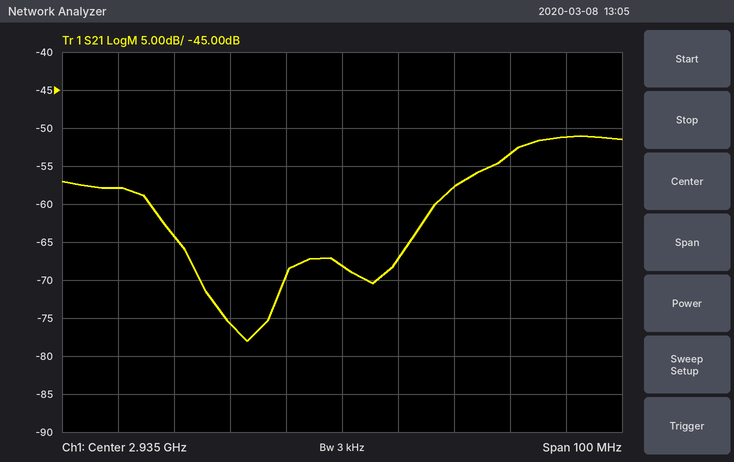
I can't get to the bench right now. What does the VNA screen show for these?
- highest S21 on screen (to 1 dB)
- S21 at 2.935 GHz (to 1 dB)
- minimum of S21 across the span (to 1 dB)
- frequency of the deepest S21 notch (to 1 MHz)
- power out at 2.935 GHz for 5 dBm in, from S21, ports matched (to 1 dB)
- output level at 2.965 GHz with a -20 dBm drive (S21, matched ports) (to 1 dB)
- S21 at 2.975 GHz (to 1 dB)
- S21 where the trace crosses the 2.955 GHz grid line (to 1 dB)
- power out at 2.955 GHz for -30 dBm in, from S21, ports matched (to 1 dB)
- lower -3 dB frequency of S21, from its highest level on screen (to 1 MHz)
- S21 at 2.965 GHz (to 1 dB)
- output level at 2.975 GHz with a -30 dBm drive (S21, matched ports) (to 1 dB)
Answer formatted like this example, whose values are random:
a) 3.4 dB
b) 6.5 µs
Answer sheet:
a) -51 dB
b) -68 dB
c) -78 dB
d) 2.918 GHz
e) -63 dBm
f) -73 dBm
g) -51 dB
h) -58 dB
i) -88 dBm
j) 2.964 GHz
k) -53 dB
l) -81 dBm
